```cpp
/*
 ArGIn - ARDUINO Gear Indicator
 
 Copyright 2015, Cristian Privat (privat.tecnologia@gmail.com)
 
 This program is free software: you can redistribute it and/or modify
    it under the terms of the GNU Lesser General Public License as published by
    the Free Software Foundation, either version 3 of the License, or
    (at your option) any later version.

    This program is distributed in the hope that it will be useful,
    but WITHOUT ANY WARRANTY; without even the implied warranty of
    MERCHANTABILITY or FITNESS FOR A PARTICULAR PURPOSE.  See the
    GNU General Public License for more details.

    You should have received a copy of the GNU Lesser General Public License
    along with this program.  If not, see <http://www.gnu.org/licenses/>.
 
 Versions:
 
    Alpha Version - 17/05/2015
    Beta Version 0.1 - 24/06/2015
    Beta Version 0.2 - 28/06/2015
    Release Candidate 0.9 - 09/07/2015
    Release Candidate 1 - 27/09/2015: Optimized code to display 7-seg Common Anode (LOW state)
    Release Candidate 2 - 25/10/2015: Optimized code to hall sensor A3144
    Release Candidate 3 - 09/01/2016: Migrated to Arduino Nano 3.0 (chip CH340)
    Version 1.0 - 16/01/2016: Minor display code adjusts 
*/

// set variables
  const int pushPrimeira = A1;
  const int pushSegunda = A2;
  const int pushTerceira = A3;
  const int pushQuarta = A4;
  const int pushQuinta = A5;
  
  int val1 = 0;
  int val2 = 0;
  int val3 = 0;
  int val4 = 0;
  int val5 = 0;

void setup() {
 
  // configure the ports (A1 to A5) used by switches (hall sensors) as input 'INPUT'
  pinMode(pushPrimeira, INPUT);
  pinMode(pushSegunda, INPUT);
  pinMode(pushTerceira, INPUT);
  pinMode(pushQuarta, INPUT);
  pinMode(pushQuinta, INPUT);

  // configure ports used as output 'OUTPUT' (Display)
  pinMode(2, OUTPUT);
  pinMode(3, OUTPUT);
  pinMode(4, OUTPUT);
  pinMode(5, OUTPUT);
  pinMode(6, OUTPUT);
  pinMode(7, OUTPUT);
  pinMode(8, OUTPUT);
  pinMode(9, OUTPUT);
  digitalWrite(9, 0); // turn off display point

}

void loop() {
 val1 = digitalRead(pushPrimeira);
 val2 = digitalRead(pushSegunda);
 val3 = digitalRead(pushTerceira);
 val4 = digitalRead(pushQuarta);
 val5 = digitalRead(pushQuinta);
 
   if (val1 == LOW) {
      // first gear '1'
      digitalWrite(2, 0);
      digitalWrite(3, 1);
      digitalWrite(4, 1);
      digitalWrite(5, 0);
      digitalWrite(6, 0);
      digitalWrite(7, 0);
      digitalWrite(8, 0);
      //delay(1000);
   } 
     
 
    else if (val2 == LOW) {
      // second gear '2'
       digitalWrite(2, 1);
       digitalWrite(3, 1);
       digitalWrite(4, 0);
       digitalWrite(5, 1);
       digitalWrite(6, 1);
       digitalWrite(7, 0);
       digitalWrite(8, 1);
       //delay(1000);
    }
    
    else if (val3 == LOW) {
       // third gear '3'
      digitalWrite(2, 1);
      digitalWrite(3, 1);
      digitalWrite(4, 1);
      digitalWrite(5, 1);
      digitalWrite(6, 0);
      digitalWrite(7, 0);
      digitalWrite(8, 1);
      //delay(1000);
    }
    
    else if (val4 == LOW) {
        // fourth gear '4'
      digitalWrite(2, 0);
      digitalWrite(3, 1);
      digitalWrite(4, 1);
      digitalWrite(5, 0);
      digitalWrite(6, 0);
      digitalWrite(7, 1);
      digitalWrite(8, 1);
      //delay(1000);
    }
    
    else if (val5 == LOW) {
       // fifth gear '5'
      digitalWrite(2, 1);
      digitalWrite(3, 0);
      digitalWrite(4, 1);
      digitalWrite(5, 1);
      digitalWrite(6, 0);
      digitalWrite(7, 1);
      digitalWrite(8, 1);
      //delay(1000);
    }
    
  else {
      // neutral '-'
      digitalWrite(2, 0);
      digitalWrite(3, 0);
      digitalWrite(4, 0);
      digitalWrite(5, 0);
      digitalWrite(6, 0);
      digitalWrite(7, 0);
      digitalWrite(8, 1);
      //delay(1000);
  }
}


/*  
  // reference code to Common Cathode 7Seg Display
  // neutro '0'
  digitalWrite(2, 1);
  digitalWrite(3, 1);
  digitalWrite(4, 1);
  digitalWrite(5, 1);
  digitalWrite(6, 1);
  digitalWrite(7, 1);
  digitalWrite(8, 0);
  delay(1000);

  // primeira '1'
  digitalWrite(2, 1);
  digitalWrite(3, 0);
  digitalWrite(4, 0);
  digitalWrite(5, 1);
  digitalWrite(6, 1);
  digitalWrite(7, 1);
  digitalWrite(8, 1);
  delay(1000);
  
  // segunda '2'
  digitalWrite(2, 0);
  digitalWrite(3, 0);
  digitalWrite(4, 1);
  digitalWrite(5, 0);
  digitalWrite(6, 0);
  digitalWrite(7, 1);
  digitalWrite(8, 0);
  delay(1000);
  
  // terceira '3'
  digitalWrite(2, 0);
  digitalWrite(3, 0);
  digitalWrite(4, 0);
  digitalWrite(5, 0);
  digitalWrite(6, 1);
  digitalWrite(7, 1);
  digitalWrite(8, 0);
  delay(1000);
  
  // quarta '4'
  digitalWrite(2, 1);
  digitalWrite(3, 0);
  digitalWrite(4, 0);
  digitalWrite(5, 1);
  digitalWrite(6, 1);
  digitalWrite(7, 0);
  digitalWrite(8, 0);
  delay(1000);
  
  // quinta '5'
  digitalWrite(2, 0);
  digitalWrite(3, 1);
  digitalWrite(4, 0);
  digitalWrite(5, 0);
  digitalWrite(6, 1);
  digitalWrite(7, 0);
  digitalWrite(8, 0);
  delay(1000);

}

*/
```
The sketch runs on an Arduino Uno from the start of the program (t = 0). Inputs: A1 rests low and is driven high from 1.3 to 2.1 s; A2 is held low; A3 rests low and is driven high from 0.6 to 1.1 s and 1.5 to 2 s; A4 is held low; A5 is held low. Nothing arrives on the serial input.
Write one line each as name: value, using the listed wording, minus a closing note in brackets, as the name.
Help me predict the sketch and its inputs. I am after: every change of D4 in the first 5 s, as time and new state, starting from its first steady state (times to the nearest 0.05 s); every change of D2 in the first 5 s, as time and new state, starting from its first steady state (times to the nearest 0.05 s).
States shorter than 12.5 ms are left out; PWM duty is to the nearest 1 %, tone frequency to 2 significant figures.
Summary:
every change of D4 in the first 5 s, as time and new state, starting from its first steady state: 0 s high; 1.3 s low; 2.1 s high
every change of D2 in the first 5 s, as time and new state, starting from its first steady state: 0 s low; 1.3 s high; 2.1 s low
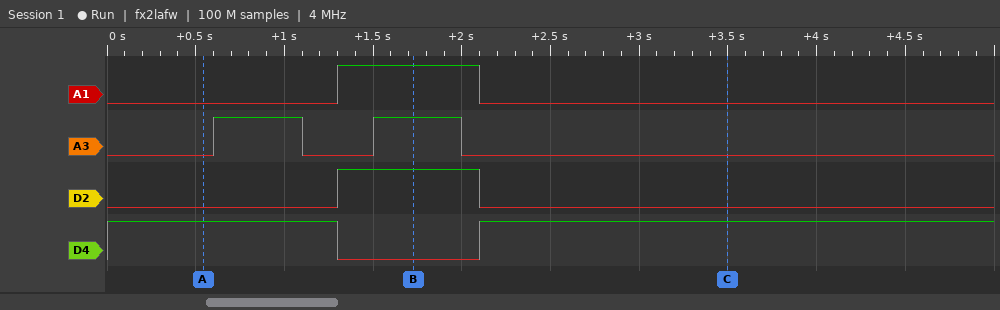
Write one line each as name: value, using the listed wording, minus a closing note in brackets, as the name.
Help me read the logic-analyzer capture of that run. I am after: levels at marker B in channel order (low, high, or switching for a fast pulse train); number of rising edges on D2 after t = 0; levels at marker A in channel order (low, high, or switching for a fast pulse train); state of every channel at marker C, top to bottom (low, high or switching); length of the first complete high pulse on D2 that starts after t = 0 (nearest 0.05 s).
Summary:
levels at marker B in channel order: A1 high, A3 high, D2 high, D4 low
number of rising edges on D2 after t = 0: 1
levels at marker A in channel order: A1 low, A3 low, D2 low, D4 high
state of every channel at marker C, top to bottom: A1 low, A3 low, D2 low, D4 high
length of the first complete high pulse on D2 that starts after t = 0: 0.80 s
